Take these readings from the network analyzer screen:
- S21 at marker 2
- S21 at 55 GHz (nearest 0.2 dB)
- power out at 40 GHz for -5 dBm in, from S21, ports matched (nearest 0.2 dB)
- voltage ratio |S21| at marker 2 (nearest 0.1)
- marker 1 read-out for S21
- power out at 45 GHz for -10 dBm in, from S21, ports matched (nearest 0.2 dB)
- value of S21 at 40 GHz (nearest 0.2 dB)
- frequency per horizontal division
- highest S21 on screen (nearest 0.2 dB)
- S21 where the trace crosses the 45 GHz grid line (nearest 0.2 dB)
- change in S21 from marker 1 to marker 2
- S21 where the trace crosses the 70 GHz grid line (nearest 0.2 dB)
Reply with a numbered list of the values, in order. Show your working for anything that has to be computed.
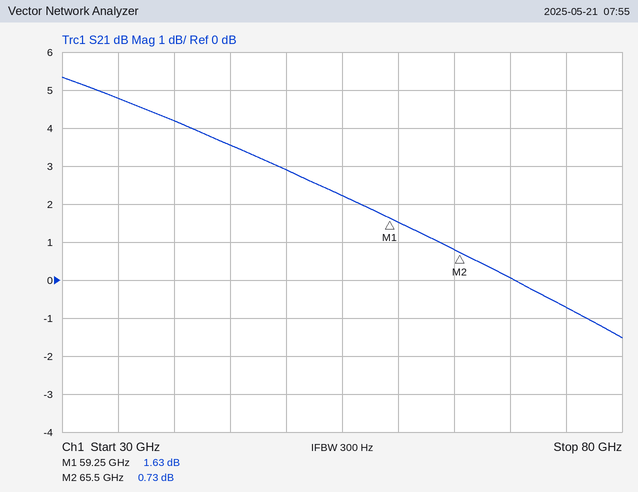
1. 0.73 dB
2. 2.2 dB
3. -5 dBm + (4.2 dB) = -0.8 dBm
4. 10^(0.73/20) ≈ 1.1
5. 1.63 dB
6. -10 dBm + (3.6 dB) = -6.4 dBm
7. 4.2 dB
8. 5 GHz
9. 5.4 dB
10. 3.6 dB
11. 0.73 − (1.63) = -0.90 dB
12. 0.0 dB
